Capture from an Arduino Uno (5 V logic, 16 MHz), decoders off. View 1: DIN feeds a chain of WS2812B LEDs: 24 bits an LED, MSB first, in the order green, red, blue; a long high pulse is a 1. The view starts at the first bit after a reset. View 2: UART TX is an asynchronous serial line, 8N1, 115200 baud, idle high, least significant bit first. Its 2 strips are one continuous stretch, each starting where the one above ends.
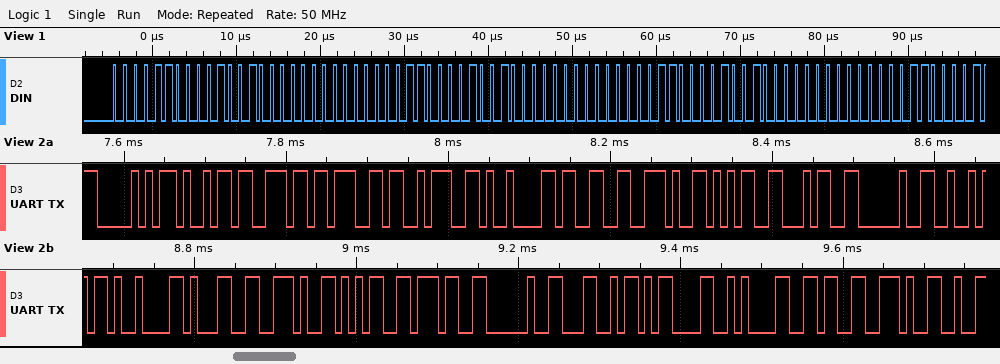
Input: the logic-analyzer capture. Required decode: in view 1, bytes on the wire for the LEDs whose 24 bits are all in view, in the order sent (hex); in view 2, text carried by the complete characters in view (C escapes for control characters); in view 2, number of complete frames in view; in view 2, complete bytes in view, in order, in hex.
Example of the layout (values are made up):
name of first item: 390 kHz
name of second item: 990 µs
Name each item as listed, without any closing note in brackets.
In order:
in view 1, bytes on the wire for the LEDs whose 24 bits are all in view, in the order sent: 0C 24 00 0C 24 00 0C 24 00
in view 2, text carried by the complete characters in view: "Ping:\t3.54 R\t1.57 L\r\n6."
in view 2, number of complete frames in view: 23
in view 2, complete bytes in view, in order, in hex: 50 69 6E 67 3A 09 33 2E 35 34 20 52 09 31 2E 35 37 20 4C 0D 0A 36 2E
